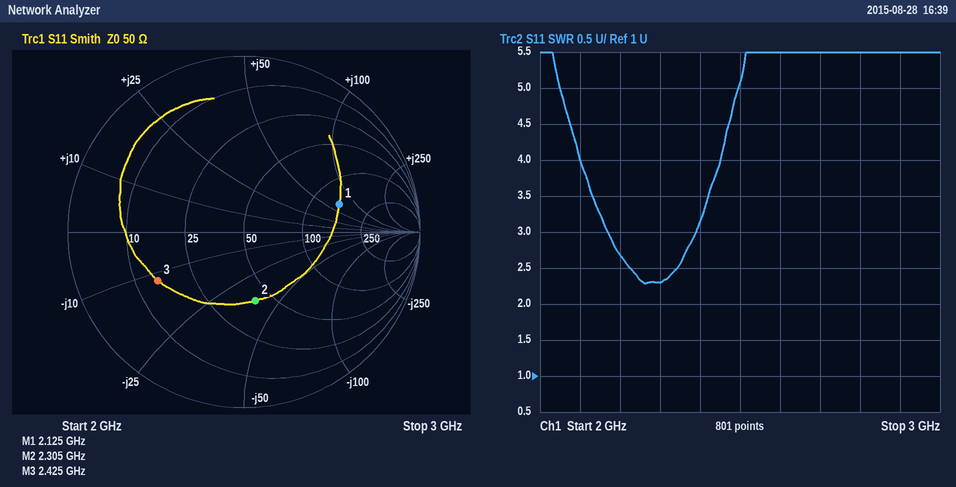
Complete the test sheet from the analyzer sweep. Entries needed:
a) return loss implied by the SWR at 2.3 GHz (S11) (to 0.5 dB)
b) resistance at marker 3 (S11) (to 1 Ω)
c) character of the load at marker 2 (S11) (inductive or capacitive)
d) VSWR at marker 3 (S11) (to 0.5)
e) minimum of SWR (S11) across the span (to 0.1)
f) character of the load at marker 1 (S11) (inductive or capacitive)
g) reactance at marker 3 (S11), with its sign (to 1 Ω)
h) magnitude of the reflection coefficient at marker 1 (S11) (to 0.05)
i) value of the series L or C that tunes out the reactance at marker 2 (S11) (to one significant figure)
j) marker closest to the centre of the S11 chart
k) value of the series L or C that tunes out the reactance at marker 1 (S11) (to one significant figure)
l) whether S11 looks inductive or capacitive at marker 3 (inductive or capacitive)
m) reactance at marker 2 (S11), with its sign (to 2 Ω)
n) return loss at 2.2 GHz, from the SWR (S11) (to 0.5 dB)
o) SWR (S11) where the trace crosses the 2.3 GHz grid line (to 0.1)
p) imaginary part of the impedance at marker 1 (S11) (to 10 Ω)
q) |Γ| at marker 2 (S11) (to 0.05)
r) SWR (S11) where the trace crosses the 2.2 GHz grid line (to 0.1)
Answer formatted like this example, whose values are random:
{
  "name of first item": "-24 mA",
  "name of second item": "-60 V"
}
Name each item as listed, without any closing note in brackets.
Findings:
{
  "return loss implied by the SWR at 2.3 GHz (S11)": "8.0 dB",
  "resistance at marker 3 (S11)": "15 Ω",
  "character of the load at marker 2 (S11)": "capacitive",
  "VSWR at marker 3 (S11)": "3.5",
  "minimum of SWR (S11) across the span": "2.3",
  "character of the load at marker 1 (S11)": "inductive",
  "reactance at marker 3 (S11), with its sign": "-12 Ω",
  "magnitude of the reflection coefficient at marker 1 (S11)": "0.55",
  "value of the series L or C that tunes out the reactance at marker 2 (S11)": "3 nH",
  "marker closest to the centre of the S11 chart": "marker 2",
  "value of the series L or C that tunes out the reactance at marker 1 (S11)": "1 pF",
  "whether S11 looks inductive or capacitive at marker 3": "capacitive",
  "reactance at marker 2 (S11), with its sign": "-38 Ω",
  "return loss at 2.2 GHz, from the SWR (S11)": "7.0 dB",
  "SWR (S11) where the trace crosses the 2.3 GHz grid line": "2.3",
  "imaginary part of the impedance at marker 1 (S11)": "+70 Ω",
  "|Γ| at marker 2 (S11)": "0.40",
  "SWR (S11) where the trace crosses the 2.2 GHz grid line": "2.7"
}
